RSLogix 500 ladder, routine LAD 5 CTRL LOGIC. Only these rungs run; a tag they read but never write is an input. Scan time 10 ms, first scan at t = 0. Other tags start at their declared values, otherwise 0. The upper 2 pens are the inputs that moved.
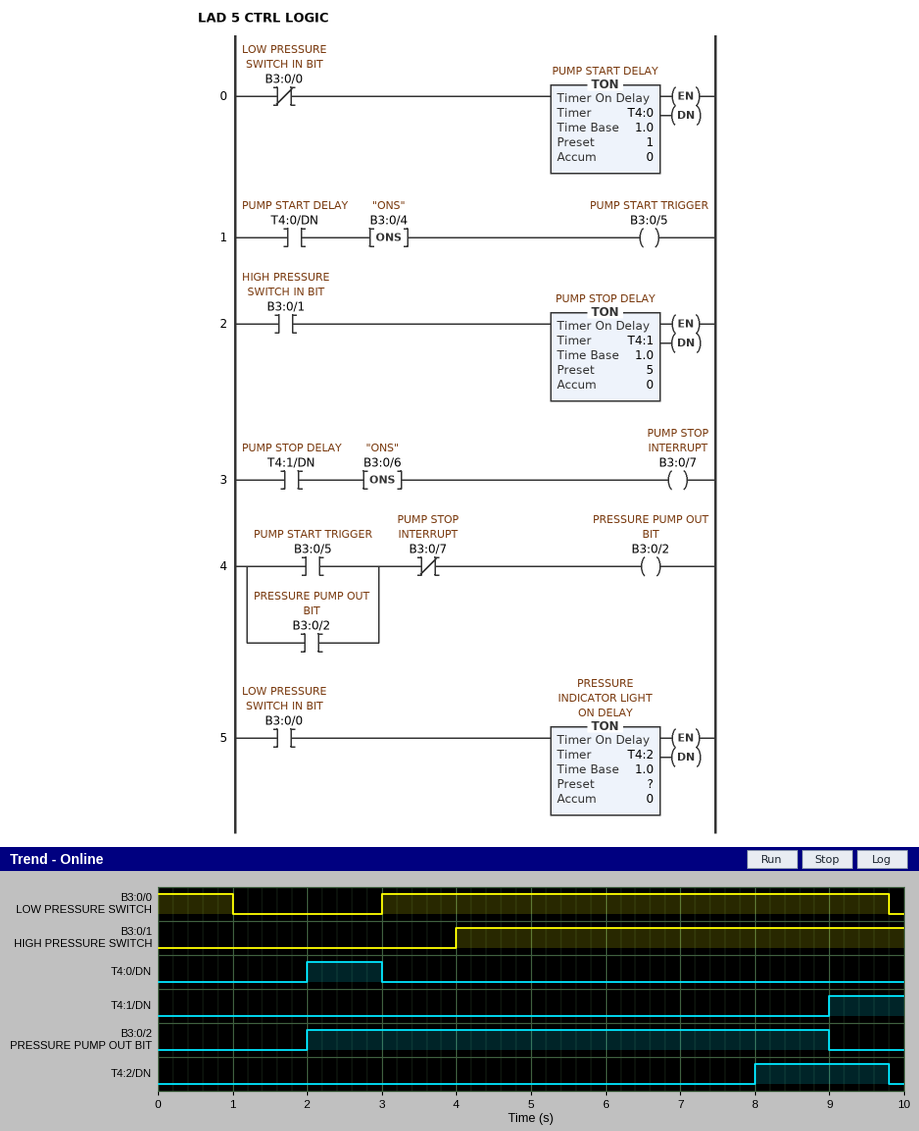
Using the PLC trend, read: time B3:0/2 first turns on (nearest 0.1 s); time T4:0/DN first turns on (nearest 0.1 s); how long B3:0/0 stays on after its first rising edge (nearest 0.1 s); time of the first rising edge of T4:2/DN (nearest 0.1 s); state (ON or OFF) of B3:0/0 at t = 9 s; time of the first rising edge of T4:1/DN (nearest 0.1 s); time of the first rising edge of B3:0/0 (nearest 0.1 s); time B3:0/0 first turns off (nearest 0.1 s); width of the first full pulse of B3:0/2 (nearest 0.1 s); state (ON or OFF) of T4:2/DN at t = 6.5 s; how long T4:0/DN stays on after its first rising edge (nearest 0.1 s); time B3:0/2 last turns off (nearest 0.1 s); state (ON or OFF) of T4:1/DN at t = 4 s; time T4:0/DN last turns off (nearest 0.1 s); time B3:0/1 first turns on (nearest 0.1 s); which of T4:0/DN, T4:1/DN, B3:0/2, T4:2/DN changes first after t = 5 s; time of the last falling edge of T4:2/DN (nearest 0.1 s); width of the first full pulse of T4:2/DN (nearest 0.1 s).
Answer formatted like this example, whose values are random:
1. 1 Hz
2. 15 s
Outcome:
1. 2.0 s
2. 2.0 s
3. 6.8 s
4. 8.0 s
5. ON
6. 9.0 s
7. 3.0 s
8. 1.0 s
9. 7.0 s
10. OFF
11. 1.0 s
12. 9.0 s
13. OFF
14. 3.0 s
15. 4.0 s
16. T4:2/DN
17. 9.8 s
18. 1.8 s
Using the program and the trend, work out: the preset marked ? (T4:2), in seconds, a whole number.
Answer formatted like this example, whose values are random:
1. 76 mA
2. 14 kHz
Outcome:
1. 5 s
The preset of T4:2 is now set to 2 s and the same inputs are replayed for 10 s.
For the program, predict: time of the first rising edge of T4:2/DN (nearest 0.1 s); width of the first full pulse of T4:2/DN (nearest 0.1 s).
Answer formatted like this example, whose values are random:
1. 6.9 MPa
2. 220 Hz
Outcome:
1. 5.0 s
2. 4.8 s
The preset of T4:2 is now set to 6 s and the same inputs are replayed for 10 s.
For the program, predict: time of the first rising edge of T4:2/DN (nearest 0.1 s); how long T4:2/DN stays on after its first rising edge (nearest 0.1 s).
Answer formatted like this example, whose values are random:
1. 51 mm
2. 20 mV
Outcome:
1. 9.0 s
2. 0.8 s
